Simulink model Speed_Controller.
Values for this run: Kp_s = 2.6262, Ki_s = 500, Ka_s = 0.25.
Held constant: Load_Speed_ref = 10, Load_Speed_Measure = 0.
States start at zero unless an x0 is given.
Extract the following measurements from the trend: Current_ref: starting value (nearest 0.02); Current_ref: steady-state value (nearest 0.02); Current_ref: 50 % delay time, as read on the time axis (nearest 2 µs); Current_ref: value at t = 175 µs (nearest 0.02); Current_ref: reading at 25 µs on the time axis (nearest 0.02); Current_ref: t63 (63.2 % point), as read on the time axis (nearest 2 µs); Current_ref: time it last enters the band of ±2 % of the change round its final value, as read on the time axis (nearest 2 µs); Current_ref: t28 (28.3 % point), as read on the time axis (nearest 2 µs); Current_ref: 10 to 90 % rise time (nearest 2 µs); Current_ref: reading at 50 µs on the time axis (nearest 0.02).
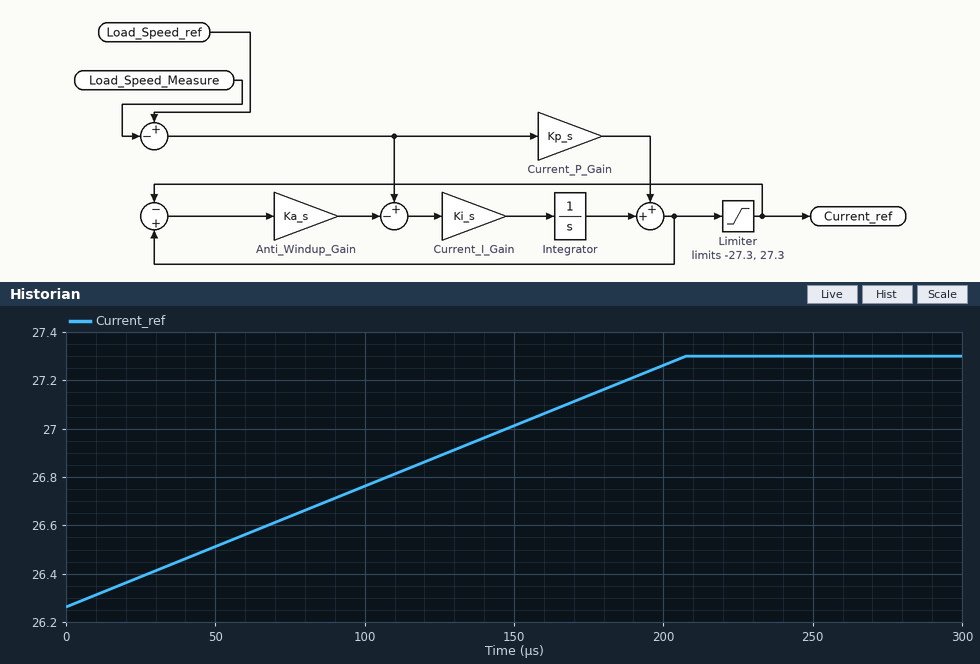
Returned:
26.26
27.30
104 µs
27.14
26.38
132 µs
204 µs
58 µs
166 µs
26.52
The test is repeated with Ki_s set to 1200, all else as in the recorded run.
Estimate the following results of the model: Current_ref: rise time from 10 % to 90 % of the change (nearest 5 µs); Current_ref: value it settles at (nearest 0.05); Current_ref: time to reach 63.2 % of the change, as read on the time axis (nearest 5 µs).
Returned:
70 µs
27.30
55 µs
